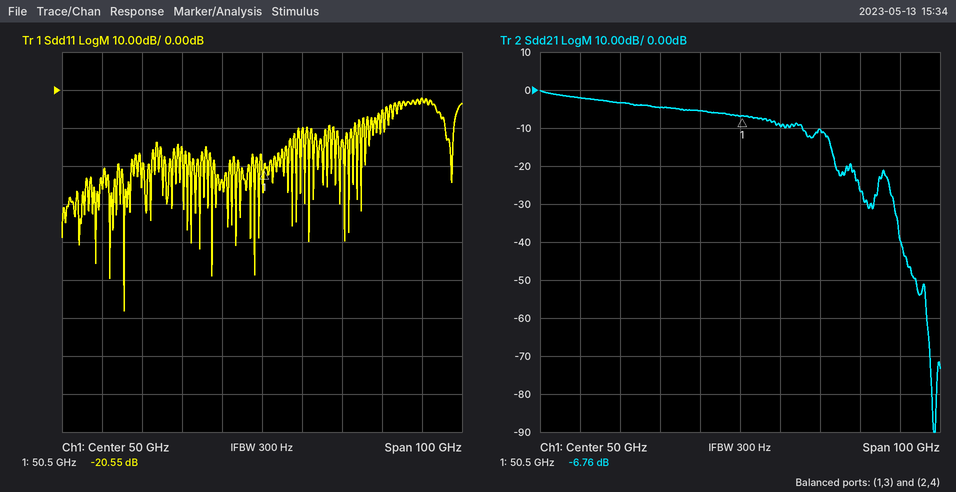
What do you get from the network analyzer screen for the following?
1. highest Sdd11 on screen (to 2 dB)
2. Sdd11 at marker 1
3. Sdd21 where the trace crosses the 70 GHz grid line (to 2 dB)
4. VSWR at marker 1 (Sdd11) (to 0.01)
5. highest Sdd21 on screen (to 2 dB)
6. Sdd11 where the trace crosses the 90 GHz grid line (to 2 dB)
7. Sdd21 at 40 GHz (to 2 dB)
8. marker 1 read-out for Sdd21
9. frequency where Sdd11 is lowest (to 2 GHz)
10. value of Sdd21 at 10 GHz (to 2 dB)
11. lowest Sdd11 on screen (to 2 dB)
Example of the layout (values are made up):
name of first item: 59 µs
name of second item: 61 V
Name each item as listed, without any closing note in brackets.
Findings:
highest Sdd11 on screen: -2 dB
Sdd11 at marker 1: -20.55 dB
Sdd21 where the trace crosses the 70 GHz grid line: -10 dB
VSWR at marker 1 (Sdd11): 1.21
highest Sdd21 on screen: 0 dB
Sdd11 where the trace crosses the 90 GHz grid line: -2 dB
Sdd21 at 40 GHz: -6 dB
marker 1 read-out for Sdd21: -6.76 dB
frequency where Sdd11 is lowest: 16 GHz
value of Sdd21 at 10 GHz: -2 dB
lowest Sdd11 on screen: -58 dB
